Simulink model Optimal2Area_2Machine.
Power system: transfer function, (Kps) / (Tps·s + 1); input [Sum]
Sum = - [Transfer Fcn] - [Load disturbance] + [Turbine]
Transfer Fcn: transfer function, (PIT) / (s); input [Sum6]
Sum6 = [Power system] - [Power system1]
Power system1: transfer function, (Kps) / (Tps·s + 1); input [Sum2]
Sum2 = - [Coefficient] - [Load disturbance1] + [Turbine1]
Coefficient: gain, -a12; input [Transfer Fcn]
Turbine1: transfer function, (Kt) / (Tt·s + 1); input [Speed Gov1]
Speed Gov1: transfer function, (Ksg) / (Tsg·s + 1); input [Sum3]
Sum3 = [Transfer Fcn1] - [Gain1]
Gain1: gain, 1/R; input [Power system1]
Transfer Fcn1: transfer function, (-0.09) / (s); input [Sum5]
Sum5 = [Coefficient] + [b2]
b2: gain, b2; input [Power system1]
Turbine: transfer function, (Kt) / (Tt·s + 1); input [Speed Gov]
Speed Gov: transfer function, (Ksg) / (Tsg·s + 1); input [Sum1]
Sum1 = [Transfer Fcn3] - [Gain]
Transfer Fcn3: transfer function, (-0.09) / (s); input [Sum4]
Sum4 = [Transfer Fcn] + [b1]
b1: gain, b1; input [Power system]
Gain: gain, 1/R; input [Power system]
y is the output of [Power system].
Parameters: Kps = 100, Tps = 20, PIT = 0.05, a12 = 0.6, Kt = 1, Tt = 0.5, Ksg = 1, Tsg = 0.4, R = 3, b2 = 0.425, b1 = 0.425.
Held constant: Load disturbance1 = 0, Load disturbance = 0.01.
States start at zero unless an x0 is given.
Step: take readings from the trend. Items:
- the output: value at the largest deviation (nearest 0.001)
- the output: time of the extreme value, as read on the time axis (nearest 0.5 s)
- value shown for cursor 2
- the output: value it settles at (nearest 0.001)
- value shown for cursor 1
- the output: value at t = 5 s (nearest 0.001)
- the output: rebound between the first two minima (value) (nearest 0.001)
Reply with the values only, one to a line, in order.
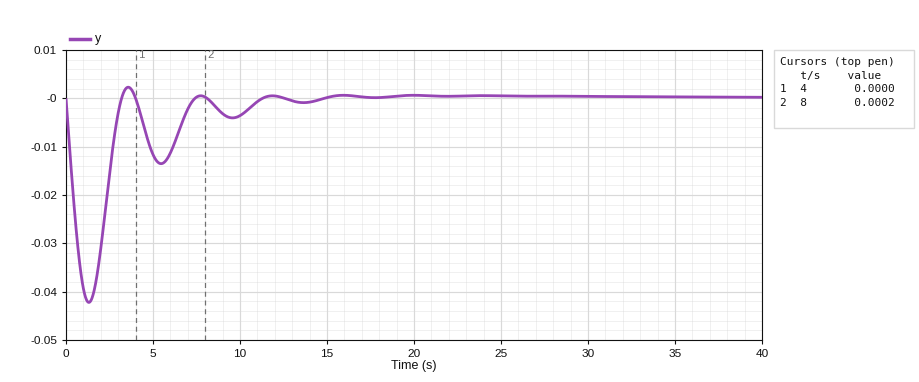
-0.042
1.5 s
0.0002
0.000
0.0000
-0.012
0.002
